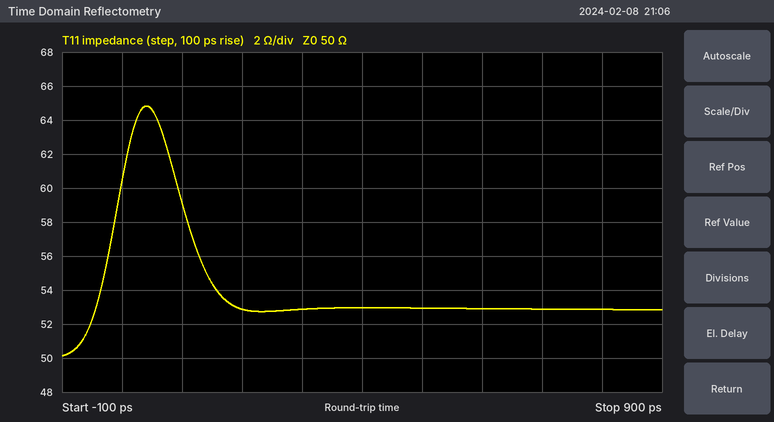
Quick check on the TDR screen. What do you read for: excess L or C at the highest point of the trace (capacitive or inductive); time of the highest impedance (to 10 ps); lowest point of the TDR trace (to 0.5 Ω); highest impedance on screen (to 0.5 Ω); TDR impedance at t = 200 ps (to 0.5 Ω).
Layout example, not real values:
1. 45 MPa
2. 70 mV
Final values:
1. inductive
2. 40 ps
3. 50.0 Ω
4. 65.0 Ω
5. 53.0 Ω
